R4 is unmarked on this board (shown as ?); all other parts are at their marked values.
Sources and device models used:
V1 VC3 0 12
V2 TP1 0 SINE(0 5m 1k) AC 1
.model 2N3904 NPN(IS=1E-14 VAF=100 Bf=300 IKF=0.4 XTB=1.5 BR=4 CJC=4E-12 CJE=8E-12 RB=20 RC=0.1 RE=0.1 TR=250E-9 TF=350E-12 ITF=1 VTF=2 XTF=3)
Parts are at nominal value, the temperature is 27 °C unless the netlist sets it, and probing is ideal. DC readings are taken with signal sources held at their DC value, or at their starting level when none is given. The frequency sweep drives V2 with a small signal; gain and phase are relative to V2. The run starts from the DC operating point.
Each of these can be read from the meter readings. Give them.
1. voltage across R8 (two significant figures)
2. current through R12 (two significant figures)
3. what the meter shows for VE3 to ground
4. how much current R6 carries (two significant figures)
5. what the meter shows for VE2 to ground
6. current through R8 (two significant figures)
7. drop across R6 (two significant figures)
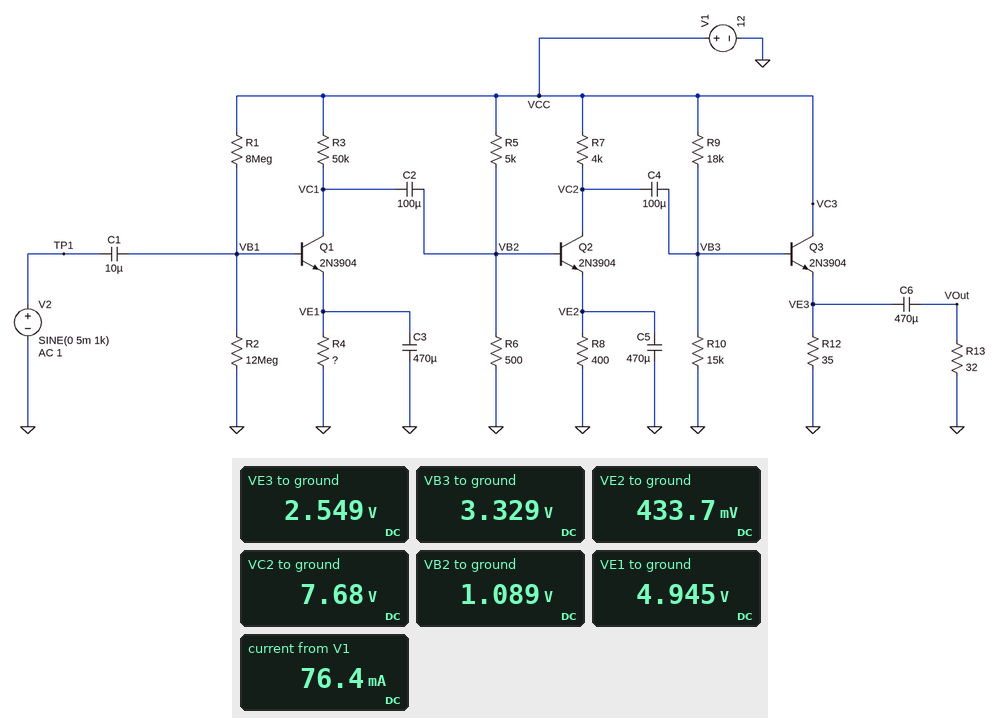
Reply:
430 mV
73 mA
2.549 V
2.2 mA
433.7 mV
1.1 mA
1.1 V
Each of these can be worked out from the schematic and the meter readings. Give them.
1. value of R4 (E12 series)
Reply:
47 kΩ
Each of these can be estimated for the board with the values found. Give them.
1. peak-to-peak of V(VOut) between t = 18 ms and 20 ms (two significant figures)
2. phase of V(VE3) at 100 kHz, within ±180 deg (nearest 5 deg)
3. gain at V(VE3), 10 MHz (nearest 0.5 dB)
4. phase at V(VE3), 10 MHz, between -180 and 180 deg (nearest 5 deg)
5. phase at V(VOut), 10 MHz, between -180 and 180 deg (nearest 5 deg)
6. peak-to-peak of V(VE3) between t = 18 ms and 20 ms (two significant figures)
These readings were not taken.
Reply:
1.1 V
-5 deg
24.0 dB
-105 deg
-105 deg
1.1 V
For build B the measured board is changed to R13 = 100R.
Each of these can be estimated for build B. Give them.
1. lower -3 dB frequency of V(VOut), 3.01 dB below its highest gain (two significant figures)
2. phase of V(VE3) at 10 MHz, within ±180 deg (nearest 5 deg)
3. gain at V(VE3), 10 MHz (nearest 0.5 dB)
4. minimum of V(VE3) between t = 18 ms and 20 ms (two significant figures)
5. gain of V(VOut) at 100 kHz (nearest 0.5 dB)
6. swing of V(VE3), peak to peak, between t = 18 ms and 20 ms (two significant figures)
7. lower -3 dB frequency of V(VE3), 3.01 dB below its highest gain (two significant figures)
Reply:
15 Hz
-100 deg
25.5 dB
1.9 V
42.0 dB
1.3 V
14 Hz
